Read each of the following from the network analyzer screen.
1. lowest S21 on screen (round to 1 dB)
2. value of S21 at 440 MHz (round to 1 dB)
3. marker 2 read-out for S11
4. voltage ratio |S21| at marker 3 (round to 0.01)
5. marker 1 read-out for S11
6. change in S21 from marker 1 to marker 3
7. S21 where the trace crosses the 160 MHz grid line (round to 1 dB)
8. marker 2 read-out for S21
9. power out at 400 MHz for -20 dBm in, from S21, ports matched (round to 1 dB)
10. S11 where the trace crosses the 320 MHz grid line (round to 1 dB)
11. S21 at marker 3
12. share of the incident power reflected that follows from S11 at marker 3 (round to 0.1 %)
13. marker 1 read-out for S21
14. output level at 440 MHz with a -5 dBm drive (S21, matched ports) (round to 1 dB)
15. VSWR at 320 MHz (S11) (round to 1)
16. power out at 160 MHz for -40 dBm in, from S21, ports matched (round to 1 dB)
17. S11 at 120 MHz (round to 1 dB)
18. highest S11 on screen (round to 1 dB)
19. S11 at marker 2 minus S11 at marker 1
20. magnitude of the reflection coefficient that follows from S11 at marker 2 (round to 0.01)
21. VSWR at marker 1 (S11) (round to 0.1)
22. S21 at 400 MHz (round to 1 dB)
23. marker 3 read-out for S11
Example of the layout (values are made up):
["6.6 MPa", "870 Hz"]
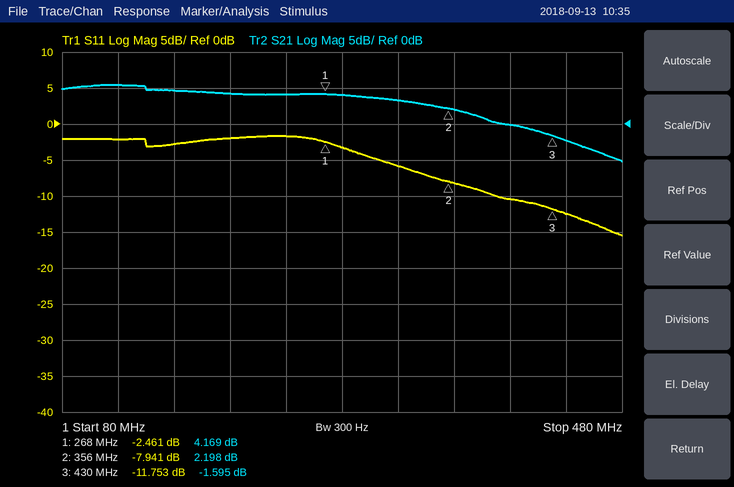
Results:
["-5 dB", "-2 dB", "-7.941 dB", "0.83", "-2.461 dB", "-5.764 dB", "5 dB", "2.198 dB", "-20 dBm", "-6 dB", "-1.595 dB", "6.7 %", "4.169 dB", "-7 dBm", "3", "-35 dBm", "-2 dB", "-2 dB", "-5.480 dB", "0.40", "7.1", "0 dB", "-11.753 dB"]
